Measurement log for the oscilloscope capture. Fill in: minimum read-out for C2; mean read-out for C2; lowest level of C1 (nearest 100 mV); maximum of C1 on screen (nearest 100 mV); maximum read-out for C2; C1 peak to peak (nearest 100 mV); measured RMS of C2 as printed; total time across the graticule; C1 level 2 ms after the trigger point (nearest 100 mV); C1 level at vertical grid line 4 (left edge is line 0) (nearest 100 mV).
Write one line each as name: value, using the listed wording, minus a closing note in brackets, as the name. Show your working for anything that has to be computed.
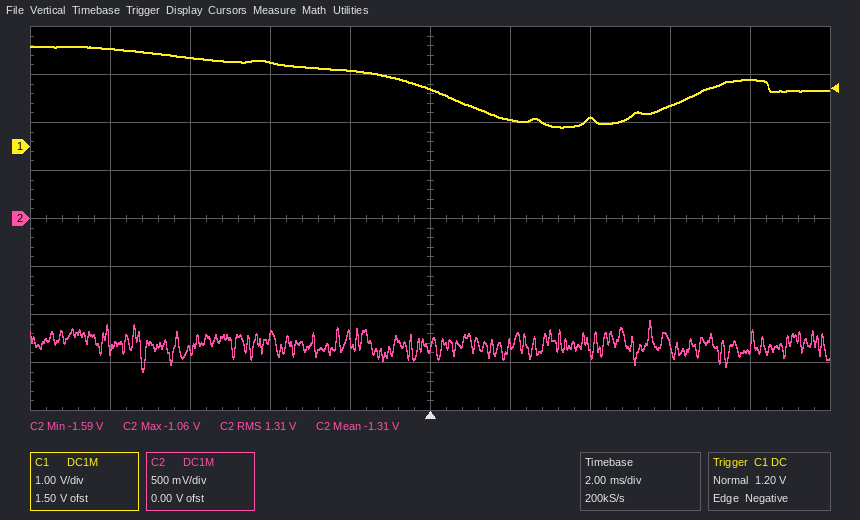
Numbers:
minimum read-out for C2: -1.59 V
mean read-out for C2: -1.31 V
lowest level of C1: 400 mV
maximum of C1 on screen: 2.1 V
maximum read-out for C2: -1.06 V
C1 peak to peak: 2.1 V − (400 mV) = 1.7 V
measured RMS of C2 as printed: 1.31 V
total time across the graticule: 20 ms
C1 level 2 ms after the trigger point: 600 mV
C1 level at vertical grid line 4 (left edge is line 0): 1.6 V
